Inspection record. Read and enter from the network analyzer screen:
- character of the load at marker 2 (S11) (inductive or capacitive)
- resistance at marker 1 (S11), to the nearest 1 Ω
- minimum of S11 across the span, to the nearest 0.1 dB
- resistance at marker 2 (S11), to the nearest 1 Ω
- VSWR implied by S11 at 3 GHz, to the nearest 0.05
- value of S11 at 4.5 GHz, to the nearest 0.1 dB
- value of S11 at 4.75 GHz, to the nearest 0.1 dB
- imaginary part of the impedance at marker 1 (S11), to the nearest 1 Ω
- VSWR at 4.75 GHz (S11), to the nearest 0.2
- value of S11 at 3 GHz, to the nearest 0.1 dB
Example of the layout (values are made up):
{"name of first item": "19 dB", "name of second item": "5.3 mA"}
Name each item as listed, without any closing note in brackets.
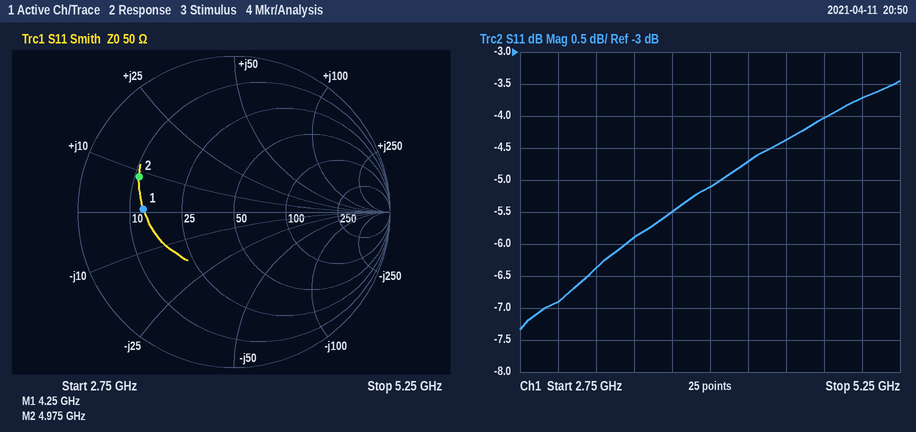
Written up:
{"character of the load at marker 2 (S11)": "inductive", "resistance at marker 1 (S11), to the nearest 1 Ω": "13 Ω", "minimum of S11 across the span, to the nearest 0.1 dB": "-7.3 dB", "resistance at marker 2 (S11), to the nearest 1 Ω": "11 Ω", "VSWR implied by S11 at 3 GHz, to the nearest 0.05": "2.65", "value of S11 at 4.5 GHz, to the nearest 0.1 dB": "-4.4 dB", "value of S11 at 4.75 GHz, to the nearest 0.1 dB": "-4.0 dB", "imaginary part of the impedance at marker 1 (S11), to the nearest 1 Ω": "+1 Ω", "VSWR at 4.75 GHz (S11), to the nearest 0.2": "4.4", "value of S11 at 3 GHz, to the nearest 0.1 dB": "-6.9 dB"}
